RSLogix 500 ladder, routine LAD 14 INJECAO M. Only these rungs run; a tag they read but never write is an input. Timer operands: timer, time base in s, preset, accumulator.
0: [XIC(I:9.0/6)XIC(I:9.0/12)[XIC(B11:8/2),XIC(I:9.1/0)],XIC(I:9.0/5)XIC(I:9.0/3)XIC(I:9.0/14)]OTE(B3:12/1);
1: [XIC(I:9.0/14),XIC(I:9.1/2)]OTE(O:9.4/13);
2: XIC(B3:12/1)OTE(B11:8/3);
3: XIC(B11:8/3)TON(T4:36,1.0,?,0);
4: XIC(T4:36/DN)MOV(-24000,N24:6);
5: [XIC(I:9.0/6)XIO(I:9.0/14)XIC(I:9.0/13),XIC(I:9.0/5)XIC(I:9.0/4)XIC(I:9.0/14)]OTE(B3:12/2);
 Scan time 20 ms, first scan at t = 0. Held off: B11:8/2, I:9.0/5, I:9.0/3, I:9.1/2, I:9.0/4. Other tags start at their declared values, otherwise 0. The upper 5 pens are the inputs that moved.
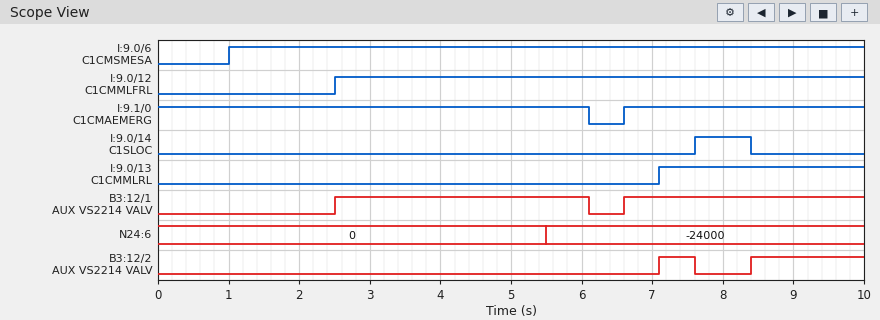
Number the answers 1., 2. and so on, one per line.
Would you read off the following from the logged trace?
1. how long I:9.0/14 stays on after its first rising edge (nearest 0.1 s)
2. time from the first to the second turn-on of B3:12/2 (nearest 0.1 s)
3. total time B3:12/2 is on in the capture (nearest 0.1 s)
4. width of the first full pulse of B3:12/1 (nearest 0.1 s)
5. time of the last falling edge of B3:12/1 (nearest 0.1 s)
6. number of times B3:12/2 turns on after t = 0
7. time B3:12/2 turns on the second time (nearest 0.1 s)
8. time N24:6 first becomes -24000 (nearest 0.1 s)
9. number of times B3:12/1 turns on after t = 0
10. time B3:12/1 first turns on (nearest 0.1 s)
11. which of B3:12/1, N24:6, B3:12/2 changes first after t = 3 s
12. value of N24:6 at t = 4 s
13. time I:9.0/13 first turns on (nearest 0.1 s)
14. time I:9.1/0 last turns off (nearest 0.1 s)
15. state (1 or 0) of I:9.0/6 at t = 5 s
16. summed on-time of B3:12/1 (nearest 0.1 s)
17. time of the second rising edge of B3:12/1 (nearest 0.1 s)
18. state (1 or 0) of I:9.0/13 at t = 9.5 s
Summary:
1. 0.8 s
2. 1.3 s
3. 2.1 s
4. 3.6 s
5. 6.1 s
6. 2
7. 8.4 s
8. 5.5 s
9. 2
10. 2.5 s
11. N24:6
12. 0
13. 7.1 s
14. 6.1 s
15. 1
16. 7.0 s
17. 6.6 s
18. 1
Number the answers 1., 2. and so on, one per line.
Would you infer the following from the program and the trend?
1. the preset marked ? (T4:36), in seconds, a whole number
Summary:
1. 3 s
